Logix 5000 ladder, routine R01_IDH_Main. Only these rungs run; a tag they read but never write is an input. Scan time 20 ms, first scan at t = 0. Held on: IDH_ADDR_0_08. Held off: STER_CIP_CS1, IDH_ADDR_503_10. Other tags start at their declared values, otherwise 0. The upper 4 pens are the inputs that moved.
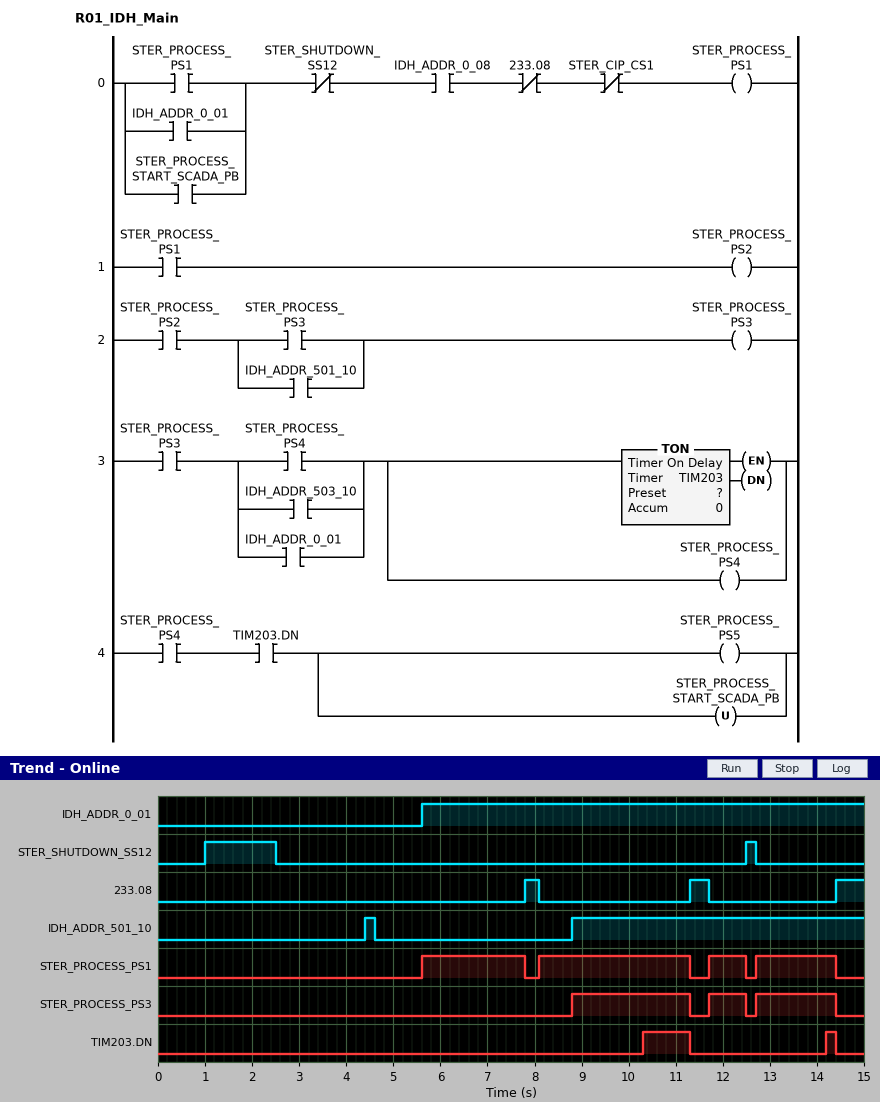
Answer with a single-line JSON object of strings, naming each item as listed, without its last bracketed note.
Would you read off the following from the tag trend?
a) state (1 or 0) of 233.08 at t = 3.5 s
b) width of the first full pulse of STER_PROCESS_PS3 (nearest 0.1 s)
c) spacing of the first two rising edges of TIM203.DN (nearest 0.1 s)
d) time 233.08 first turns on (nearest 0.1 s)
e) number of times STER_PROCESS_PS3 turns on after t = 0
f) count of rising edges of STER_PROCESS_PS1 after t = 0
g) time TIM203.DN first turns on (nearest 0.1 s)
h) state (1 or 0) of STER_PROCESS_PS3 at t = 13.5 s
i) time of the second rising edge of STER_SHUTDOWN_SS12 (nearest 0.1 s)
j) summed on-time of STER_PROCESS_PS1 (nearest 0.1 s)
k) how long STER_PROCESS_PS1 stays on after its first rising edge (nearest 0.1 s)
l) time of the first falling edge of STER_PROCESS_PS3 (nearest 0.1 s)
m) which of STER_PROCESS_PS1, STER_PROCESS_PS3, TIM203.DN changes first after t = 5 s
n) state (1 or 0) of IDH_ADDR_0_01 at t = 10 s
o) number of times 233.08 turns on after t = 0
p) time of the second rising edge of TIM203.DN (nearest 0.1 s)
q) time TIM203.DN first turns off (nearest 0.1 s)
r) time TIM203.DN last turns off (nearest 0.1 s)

{"state (1 or 0) of 233.08 at t = 3.5 s": "0", "width of the first full pulse of STER_PROCESS_PS3": "2.5 s", "spacing of the first two rising edges of TIM203.DN": "3.9 s", "time 233.08 first turns on": "7.8 s", "number of times STER_PROCESS_PS3 turns on after t = 0": "3", "count of rising edges of STER_PROCESS_PS1 after t = 0": "4", "time TIM203.DN first turns on": "10.3 s", "state (1 or 0) of STER_PROCESS_PS3 at t = 13.5 s": "1", "time of the second rising edge of STER_SHUTDOWN_SS12": "12.5 s", "summed on-time of STER_PROCESS_PS1": "7.9 s", "how long STER_PROCESS_PS1 stays on after its first rising edge": "2.2 s", "time of the first falling edge of STER_PROCESS_PS3": "11.3 s", "which of STER_PROCESS_PS1, STER_PROCESS_PS3, TIM203.DN changes first after t = 5 s": "STER_PROCESS_PS1", "state (1 or 0) of IDH_ADDR_0_01 at t = 10 s": "1", "number of times 233.08 turns on after t = 0": "3", "time of the second rising edge of TIM203.DN": "14.2 s", "time TIM203.DN first turns off": "11.3 s", "time TIM203.DN last turns off": "14.4 s"}
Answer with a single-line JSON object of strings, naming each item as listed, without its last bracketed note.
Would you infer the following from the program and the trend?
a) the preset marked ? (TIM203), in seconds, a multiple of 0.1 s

{"the preset marked ? (TIM203), in seconds, a multiple of 0.1 s": "1.5 s"}
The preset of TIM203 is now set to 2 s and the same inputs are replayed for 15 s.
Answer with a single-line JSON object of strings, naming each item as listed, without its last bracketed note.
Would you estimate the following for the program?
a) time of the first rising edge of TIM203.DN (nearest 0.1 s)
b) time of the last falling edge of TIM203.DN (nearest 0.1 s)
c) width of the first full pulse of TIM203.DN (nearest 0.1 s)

{"time of the first rising edge of TIM203.DN": "10.8 s", "time of the last falling edge of TIM203.DN": "11.3 s", "width of the first full pulse of TIM203.DN": "0.5 s"}
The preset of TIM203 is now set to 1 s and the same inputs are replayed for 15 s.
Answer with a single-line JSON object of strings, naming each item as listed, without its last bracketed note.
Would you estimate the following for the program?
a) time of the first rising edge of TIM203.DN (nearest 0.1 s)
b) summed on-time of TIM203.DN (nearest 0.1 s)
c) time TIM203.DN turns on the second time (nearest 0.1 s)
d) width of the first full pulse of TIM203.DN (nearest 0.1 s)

{"time of the first rising edge of TIM203.DN": "9.8 s", "summed on-time of TIM203.DN": "2.2 s", "time TIM203.DN turns on the second time": "13.7 s", "width of the first full pulse of TIM203.DN": "1.5 s"}
